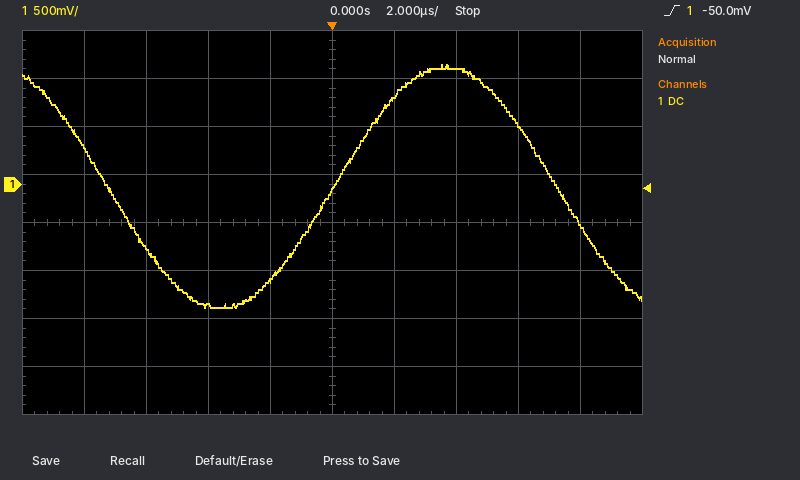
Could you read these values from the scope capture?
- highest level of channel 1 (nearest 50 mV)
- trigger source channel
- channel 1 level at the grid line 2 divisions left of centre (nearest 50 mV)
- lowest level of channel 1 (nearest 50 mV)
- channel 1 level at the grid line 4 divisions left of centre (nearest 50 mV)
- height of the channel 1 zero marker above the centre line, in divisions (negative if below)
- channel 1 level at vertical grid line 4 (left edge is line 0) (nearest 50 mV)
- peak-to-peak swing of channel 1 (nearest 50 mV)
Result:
1.25 V
channel 1
-1.25 V
-1.30 V
400 mV
+0.8 div
-1.00 V
2.55 V
